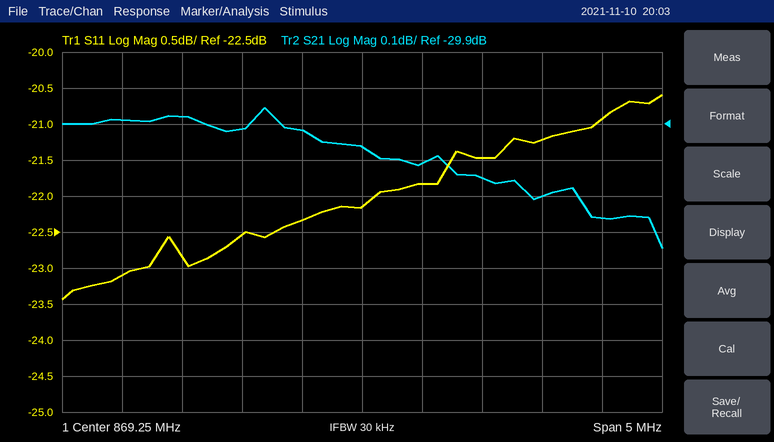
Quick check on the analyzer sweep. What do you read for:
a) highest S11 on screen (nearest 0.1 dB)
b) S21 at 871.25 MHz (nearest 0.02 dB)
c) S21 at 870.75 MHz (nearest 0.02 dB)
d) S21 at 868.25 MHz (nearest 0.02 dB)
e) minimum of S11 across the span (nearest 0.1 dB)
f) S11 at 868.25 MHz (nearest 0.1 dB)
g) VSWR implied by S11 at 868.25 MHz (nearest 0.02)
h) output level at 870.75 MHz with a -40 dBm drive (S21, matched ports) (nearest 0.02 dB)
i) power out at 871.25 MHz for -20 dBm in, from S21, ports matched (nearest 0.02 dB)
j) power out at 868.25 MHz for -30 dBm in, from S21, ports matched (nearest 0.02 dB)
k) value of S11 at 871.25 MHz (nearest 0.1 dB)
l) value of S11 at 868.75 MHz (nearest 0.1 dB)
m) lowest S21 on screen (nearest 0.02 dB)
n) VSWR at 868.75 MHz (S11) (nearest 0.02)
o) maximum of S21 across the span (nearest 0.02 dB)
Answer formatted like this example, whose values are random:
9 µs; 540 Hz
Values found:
-20.6 dB; -30.16 dB; -30.10 dB; -29.92 dB; -23.4 dB; -22.5 dB; 1.16; -70.10 dBm; -50.16 dBm; -59.92 dBm; -20.9 dB; -22.3 dB; -30.24 dB; 1.16; -29.86 dB
